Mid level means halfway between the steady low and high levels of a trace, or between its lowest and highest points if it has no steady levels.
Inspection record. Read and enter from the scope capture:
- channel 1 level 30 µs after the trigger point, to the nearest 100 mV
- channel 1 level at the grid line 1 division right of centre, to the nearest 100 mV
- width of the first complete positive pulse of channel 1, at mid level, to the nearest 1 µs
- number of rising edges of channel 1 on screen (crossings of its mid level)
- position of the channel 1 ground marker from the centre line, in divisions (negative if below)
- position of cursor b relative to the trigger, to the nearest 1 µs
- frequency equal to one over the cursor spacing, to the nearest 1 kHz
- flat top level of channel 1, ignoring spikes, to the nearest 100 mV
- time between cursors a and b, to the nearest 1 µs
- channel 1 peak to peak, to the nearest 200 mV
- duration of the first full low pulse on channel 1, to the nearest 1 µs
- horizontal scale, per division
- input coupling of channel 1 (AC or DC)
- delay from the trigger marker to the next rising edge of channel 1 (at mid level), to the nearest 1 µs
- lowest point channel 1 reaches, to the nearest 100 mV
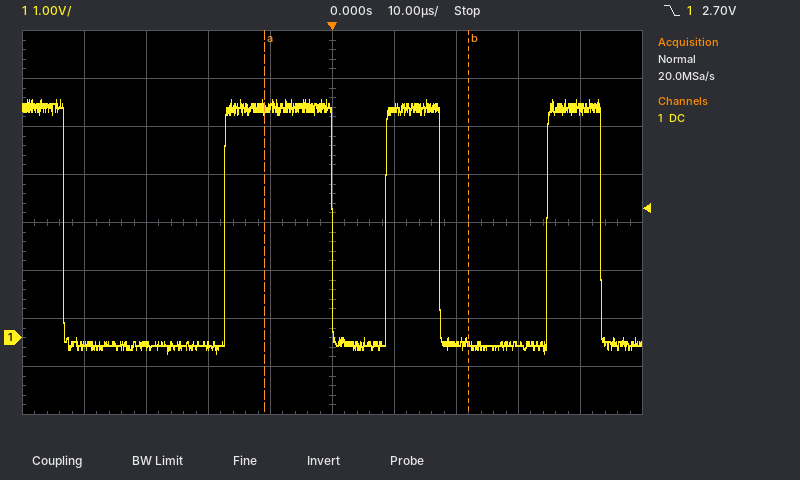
-100 mV
4.8 V
17 µs
3
-2.4 div
+22 µs
30 kHz
4.8 V
33 µs
5.2 V
26 µs
10 µs
DC
9 µs
-300 mV
